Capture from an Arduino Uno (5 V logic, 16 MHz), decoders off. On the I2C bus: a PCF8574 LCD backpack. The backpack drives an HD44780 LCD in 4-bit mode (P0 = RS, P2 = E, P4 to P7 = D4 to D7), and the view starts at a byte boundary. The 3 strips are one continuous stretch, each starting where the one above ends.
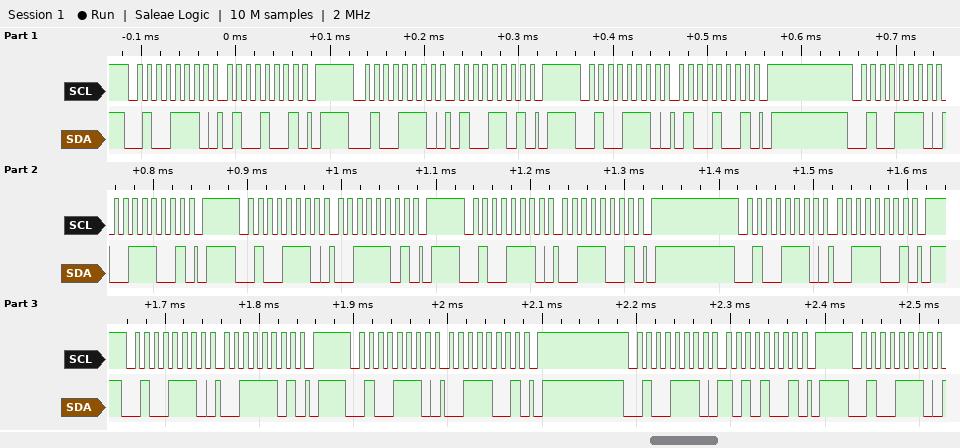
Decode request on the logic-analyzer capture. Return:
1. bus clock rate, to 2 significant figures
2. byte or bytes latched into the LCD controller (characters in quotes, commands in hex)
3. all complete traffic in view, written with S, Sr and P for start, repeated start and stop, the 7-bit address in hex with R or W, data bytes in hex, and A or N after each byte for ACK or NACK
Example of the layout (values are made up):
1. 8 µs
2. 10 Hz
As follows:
1. 100 kHz
2. 'C'
3. S 27W A 49 A P S 27W A 4D A P S 27W A 49 A P S 27W A 39 A P S 27W A 3D A P S 27W A 39 A P S 27W A 39 A P S 27W A 3D A P S 27W A 39 A P S 27W A A9 A P S 27W A
